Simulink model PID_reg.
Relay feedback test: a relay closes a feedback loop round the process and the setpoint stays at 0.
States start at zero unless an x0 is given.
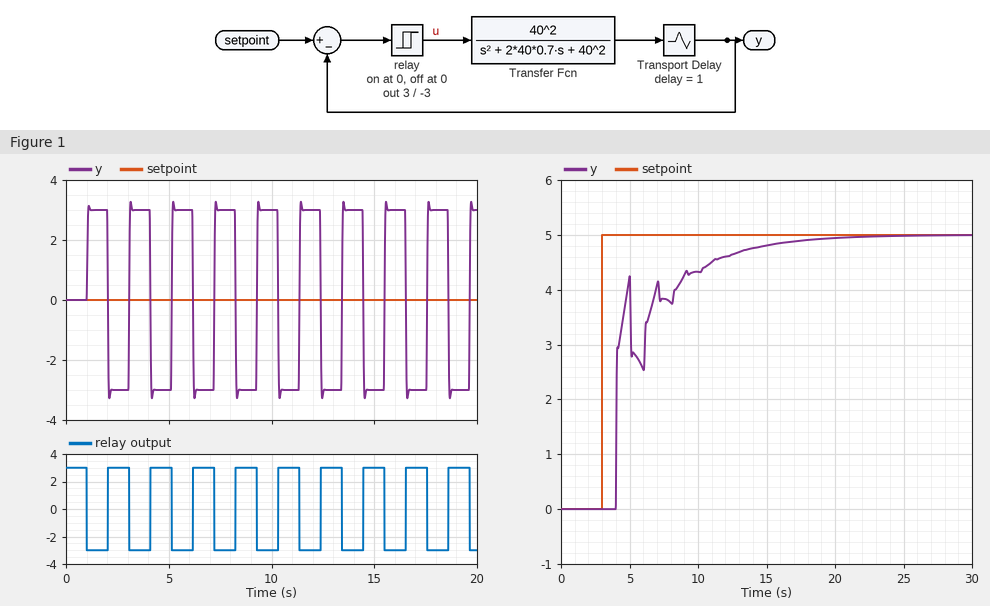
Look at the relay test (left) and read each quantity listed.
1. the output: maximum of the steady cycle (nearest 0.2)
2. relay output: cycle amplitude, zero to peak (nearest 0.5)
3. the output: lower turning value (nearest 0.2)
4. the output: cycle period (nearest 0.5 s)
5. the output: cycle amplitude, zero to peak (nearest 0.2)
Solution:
3.2
3.0
-3.2
2.0 s
3.2
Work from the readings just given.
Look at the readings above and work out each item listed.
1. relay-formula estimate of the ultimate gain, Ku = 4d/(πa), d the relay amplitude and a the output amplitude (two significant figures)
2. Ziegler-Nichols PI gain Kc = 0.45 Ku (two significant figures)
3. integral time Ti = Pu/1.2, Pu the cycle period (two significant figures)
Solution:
1.2
0.54
1.7 s
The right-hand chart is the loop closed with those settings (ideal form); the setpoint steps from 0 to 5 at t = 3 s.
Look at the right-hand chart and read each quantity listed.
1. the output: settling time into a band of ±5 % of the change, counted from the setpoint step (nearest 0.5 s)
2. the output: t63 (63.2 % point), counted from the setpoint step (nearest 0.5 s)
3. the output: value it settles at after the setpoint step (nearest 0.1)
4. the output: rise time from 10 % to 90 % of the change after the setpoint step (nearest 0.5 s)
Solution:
11.0 s
1.5 s
5.0
7.0 s
